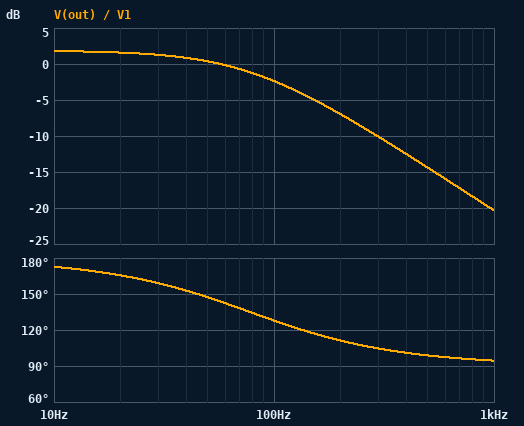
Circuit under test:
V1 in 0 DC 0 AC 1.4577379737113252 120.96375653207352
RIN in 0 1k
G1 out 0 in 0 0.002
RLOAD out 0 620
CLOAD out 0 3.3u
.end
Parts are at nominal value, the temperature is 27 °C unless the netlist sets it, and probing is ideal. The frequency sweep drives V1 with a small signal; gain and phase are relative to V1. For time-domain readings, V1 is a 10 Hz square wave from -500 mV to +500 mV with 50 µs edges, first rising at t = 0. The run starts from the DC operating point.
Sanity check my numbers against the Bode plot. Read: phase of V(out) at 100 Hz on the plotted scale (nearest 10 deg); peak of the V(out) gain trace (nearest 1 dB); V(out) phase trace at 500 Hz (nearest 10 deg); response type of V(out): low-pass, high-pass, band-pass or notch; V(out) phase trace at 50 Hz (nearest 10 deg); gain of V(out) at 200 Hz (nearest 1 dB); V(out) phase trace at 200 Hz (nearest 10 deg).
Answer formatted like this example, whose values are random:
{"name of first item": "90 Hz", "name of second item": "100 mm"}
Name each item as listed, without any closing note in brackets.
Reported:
{"phase of V(out) at 100 Hz on the plotted scale": "130 deg", "peak of the V(out) gain trace": "2 dB", "V(out) phase trace at 500 Hz": "100 deg", "response type of V(out): low-pass, high-pass, band-pass or notch": "low-pass", "V(out) phase trace at 50 Hz": "150 deg", "gain of V(out) at 200 Hz": "-7 dB", "V(out) phase trace at 200 Hz": "110 deg"}
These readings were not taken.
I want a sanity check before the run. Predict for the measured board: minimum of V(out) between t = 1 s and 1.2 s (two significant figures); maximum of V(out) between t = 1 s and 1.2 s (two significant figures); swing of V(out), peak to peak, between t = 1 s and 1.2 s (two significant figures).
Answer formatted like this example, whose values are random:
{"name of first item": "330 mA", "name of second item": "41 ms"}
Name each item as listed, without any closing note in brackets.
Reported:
{"minimum of V(out) between t = 1 s and 1.2 s": "-620 mV", "maximum of V(out) between t = 1 s and 1.2 s": "620 mV", "swing of V(out), peak to peak, between t = 1 s and 1.2 s": "1.2 V"}
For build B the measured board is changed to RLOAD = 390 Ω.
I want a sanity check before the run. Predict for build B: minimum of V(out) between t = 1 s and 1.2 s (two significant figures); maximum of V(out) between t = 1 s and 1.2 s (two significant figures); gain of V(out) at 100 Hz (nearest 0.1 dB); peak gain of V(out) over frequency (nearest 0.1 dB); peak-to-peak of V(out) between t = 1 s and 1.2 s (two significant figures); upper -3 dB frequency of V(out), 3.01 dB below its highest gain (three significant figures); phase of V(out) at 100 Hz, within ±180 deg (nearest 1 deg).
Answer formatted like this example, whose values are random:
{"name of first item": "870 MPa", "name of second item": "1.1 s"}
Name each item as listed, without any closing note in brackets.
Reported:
{"minimum of V(out) between t = 1 s and 1.2 s": "-390 mV", "maximum of V(out) between t = 1 s and 1.2 s": "390 mV", "gain of V(out) at 100 Hz": "-4.3 dB", "peak gain of V(out) over frequency": "-2.2 dB", "peak-to-peak of V(out) between t = 1 s and 1.2 s": "780 mV", "upper -3 dB frequency of V(out), 3.01 dB below its highest gain": "124 Hz", "phase of V(out) at 100 Hz, within ±180 deg": "141 deg"}
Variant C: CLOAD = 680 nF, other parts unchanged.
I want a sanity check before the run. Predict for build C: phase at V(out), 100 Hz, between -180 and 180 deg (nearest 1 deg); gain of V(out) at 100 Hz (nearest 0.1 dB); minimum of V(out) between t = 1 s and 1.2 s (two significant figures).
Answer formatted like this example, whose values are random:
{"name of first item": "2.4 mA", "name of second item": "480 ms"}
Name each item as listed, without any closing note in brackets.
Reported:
{"phase at V(out), 100 Hz, between -180 and 180 deg": "165 deg", "gain of V(out) at 100 Hz": "1.6 dB", "minimum of V(out) between t = 1 s and 1.2 s": "-620 mV"}
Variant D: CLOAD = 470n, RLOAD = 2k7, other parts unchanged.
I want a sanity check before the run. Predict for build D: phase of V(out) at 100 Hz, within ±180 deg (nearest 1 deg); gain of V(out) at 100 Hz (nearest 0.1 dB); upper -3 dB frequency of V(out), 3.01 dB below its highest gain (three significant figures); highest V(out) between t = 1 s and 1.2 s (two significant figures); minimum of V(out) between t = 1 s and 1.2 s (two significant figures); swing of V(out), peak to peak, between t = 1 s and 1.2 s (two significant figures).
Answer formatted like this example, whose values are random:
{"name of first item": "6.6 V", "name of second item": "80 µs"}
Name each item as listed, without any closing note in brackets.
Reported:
{"phase of V(out) at 100 Hz, within ±180 deg": "141 deg", "gain of V(out) at 100 Hz": "12.5 dB", "upper -3 dB frequency of V(out), 3.01 dB below its highest gain": "125 Hz", "highest V(out) between t = 1 s and 1.2 s": "2.7 V", "minimum of V(out) between t = 1 s and 1.2 s": "-2.7 V", "swing of V(out), peak to peak, between t = 1 s and 1.2 s": "5.4 V"}
